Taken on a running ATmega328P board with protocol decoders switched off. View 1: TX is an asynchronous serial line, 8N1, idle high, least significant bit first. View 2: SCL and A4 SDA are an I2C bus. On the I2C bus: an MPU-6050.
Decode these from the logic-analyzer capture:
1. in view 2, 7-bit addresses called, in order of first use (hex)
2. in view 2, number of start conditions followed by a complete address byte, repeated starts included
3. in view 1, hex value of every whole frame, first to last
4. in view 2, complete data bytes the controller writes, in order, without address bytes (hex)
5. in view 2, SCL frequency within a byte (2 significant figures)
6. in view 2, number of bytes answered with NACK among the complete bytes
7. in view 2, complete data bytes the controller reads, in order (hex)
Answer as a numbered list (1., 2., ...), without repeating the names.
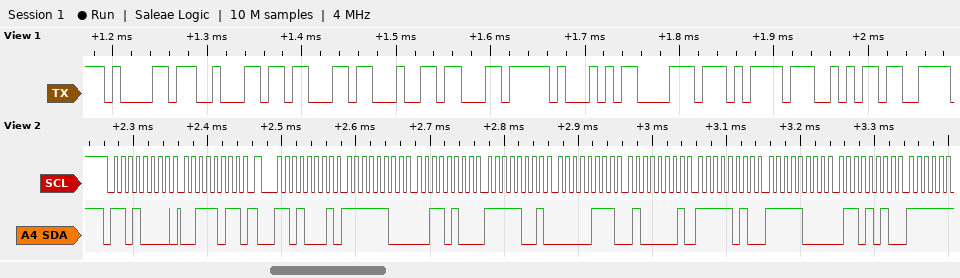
1. 0x68
2. 2
3. 0x61 0x62 0x63 0x64 0xEC 0x51 0xB8 0xBD 0x6A
4. 3B
5. 100 kHz
6. 0
7. FC 34 F9 07 41 FA F8 6A
